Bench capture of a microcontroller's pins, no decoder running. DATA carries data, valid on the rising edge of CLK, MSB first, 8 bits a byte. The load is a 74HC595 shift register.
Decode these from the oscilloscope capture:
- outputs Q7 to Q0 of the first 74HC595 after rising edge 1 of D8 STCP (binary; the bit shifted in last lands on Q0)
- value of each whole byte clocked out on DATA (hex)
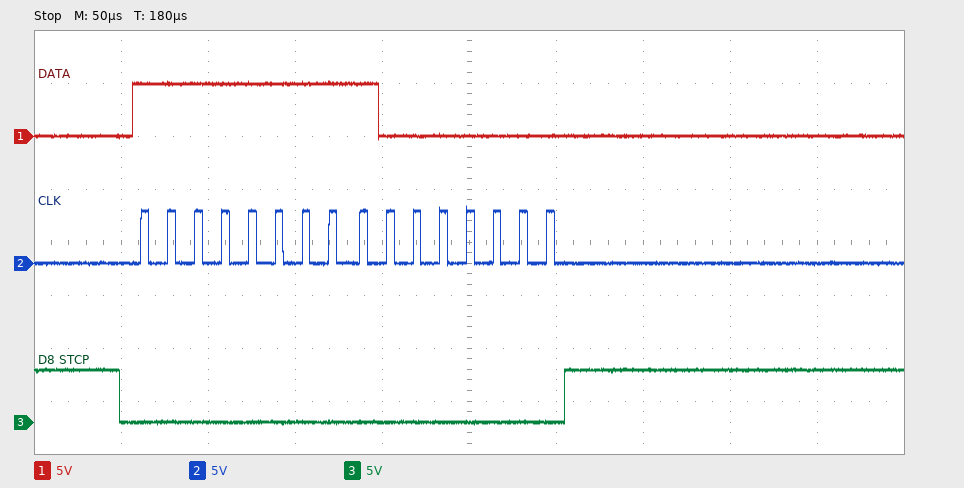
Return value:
10000000
FF 80
